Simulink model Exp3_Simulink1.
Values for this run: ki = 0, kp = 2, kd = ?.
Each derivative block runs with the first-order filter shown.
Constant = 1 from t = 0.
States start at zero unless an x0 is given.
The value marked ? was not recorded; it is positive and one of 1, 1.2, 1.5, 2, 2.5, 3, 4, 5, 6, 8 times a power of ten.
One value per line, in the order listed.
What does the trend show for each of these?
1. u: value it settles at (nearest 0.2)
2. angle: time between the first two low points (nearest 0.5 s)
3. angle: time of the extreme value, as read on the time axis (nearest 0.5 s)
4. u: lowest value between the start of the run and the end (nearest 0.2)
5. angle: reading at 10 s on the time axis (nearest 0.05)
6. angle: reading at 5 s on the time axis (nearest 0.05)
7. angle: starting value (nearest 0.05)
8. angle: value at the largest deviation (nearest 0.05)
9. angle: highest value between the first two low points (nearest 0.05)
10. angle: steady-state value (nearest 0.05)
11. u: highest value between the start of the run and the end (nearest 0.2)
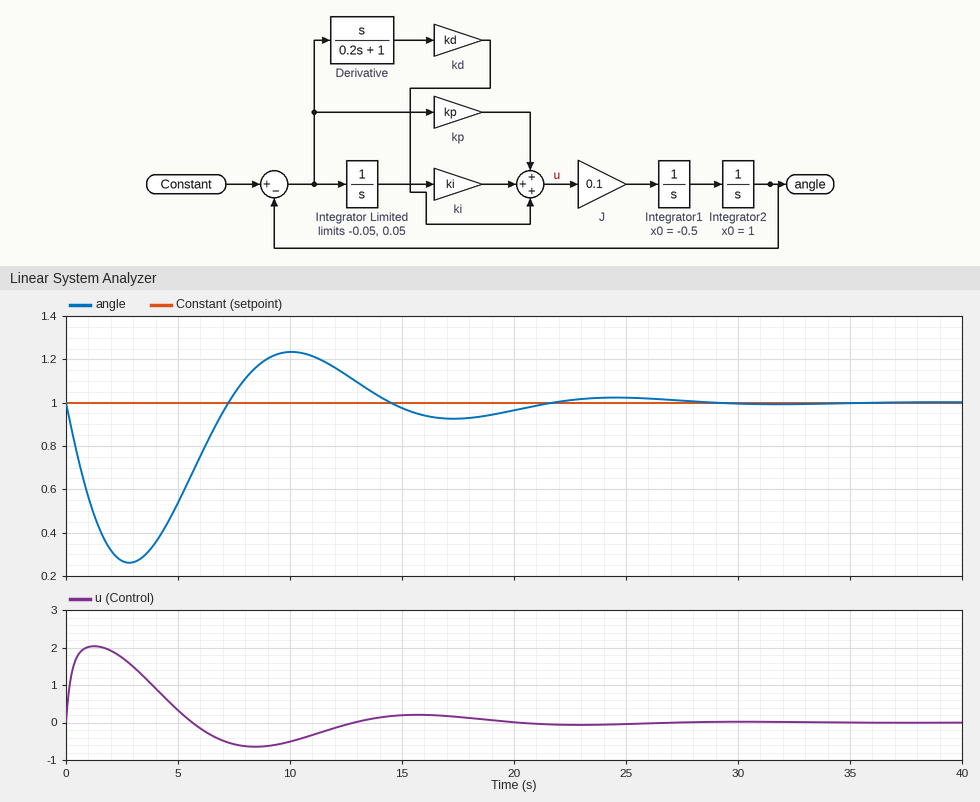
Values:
0.0
14.5 s
3.0 s
-0.6
1.25
0.55
1.00
0.25
1.25
1.00
2.0
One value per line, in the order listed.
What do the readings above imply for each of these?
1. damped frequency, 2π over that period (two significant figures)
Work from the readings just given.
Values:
0.43 rad/s
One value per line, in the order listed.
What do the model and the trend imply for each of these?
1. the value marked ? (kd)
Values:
3
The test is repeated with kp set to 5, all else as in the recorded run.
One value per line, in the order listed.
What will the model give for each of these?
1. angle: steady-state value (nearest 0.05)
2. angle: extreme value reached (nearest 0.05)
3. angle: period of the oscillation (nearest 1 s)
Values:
1.00
0.45
9 s
